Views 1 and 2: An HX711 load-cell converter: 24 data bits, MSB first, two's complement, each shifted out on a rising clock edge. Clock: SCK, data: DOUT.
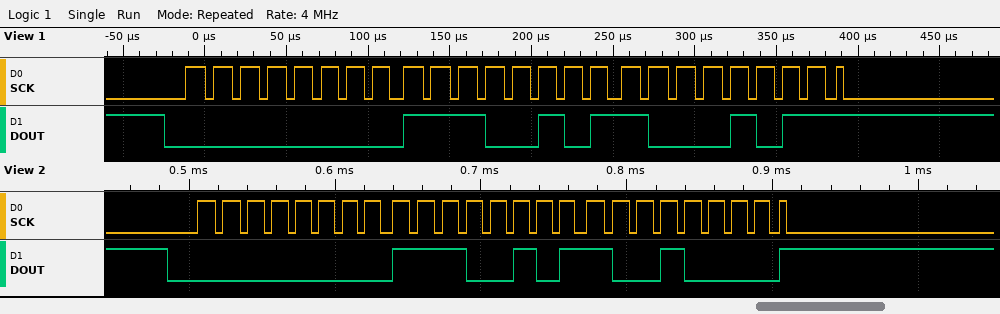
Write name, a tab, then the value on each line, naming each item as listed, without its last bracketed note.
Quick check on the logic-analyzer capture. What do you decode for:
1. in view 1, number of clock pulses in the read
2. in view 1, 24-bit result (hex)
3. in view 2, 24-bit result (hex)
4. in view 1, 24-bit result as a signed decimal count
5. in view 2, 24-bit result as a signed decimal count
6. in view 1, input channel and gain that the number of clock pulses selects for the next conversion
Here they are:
in view 1, number of clock pulses in the read	25
in view 1, 24-bit result	0x00E58B
in view 2, 24-bit result	0x00E590
in view 1, 24-bit result as a signed decimal count	58763
in view 2, 24-bit result as a signed decimal count	58768
in view 1, input channel and gain that the number of clock pulses selects for the next conversion	channel A, gain 128
